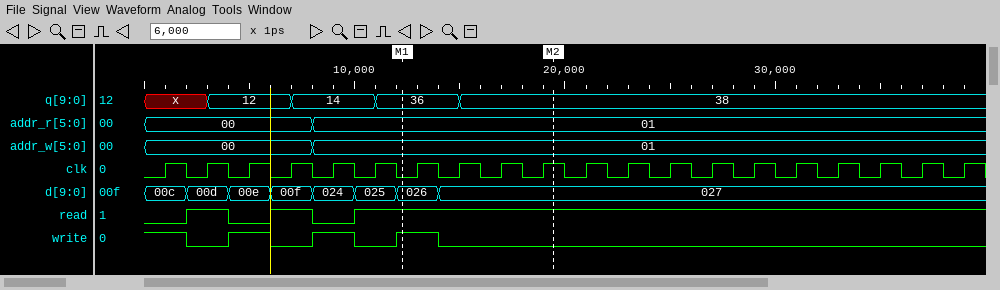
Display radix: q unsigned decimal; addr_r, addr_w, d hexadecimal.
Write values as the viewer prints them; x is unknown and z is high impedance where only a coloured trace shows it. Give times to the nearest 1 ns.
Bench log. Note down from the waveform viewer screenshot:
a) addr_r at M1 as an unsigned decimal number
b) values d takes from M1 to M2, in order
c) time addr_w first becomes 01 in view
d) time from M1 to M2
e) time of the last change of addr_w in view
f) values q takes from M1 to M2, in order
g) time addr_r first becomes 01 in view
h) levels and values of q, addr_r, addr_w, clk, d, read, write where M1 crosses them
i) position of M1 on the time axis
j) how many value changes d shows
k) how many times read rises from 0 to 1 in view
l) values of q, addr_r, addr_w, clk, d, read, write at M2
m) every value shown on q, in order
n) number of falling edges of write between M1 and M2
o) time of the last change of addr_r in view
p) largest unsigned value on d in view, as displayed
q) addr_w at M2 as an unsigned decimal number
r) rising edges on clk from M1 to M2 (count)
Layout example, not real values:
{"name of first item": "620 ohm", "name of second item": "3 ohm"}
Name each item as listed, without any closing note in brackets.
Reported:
{"addr_r at M1 as an unsigned decimal number": "1", "values d takes from M1 to M2, in order": "026, 027", "time addr_w first becomes 01 in view": "8 ns", "time from M1 to M2": "7 ns", "time of the last change of addr_w in view": "8 ns", "values q takes from M1 to M2, in order": "36, 38", "time addr_r first becomes 01 in view": "8 ns", "levels and values of q, addr_r, addr_w, clk, d, read, write where M1 crosses them": "q=36, addr_r=01, addr_w=01, clk=0, d=026, read=1, write=1", "position of M1 on the time axis": "12 ns", "how many value changes d shows": "7", "how many times read rises from 0 to 1 in view": "3", "values of q, addr_r, addr_w, clk, d, read, write at M2": "q=38, addr_r=01, addr_w=01, clk=1, d=027, read=1, write=0", "every value shown on q, in order": "x, 12, 14, 36, 38", "number of falling edges of write between M1 and M2": "1", "time of the last change of addr_r in view": "8 ns", "largest unsigned value on d in view, as displayed": "027", "addr_w at M2 as an unsigned decimal number": "1", "rising edges on clk from M1 to M2": "4"}
